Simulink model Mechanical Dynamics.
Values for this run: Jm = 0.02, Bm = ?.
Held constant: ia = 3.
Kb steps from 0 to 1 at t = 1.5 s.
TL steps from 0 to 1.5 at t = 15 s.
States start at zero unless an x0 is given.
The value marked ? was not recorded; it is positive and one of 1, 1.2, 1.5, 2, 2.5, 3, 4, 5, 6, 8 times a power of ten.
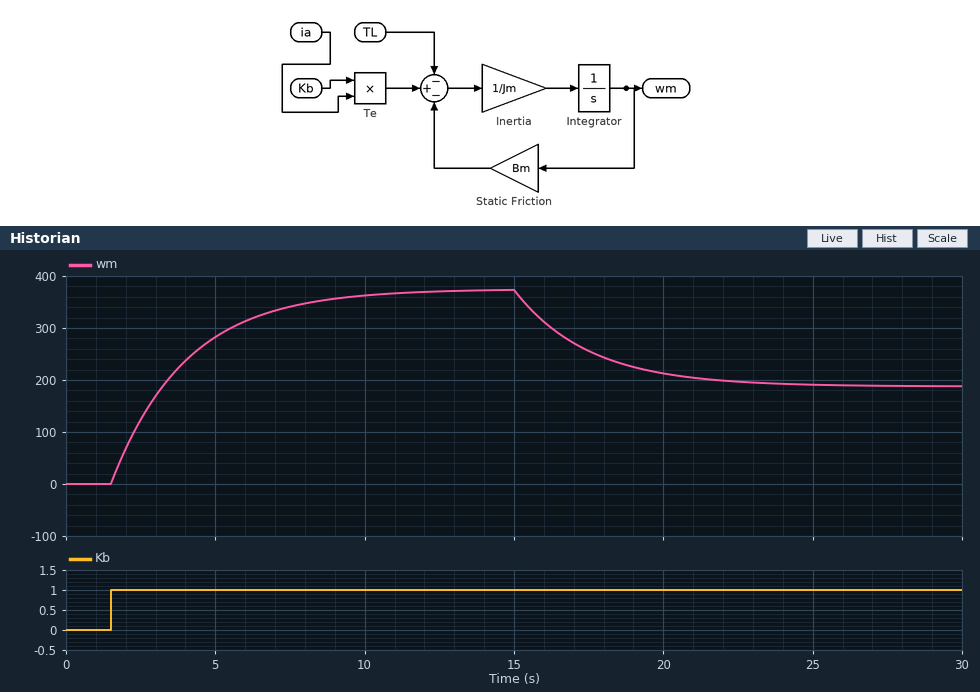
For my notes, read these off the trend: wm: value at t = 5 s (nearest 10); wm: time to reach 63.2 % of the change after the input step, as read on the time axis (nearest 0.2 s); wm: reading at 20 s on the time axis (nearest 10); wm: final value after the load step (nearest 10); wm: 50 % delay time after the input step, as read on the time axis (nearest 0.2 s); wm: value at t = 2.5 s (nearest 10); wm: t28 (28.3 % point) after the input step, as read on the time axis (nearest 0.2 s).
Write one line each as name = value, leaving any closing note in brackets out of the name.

wm: value at t = 5 s = 280
wm: time to reach 63.2 % of the change after the input step, as read on the time axis = 4.0 s
wm: reading at 20 s on the time axis = 210
wm: final value after the load step = 190
wm: 50 % delay time after the input step, as read on the time axis = 3.2 s
wm: value at t = 2.5 s = 120
wm: t28 (28.3 % point) after the input step, as read on the time axis = 2.4 s
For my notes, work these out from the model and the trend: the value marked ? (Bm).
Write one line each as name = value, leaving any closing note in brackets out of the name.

the value marked ? = 0.008
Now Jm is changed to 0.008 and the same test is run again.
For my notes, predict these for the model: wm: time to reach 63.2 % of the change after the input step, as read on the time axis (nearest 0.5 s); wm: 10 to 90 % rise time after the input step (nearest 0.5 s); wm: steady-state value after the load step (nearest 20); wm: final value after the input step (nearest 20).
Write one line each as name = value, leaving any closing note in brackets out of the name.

wm: time to reach 63.2 % of the change after the input step, as read on the time axis = 2.5 s
wm: 10 to 90 % rise time after the input step = 2.0 s
wm: steady-state value after the load step = 180
wm: final value after the input step = 380
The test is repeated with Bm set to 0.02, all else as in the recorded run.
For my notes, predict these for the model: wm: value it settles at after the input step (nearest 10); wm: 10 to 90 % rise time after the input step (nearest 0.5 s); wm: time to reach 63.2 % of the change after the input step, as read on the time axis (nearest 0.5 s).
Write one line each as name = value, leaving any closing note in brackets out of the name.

wm: value it settles at after the input step = 150
wm: 10 to 90 % rise time after the input step = 2.0 s
wm: time to reach 63.2 % of the change after the input step, as read on the time axis = 2.5 s
